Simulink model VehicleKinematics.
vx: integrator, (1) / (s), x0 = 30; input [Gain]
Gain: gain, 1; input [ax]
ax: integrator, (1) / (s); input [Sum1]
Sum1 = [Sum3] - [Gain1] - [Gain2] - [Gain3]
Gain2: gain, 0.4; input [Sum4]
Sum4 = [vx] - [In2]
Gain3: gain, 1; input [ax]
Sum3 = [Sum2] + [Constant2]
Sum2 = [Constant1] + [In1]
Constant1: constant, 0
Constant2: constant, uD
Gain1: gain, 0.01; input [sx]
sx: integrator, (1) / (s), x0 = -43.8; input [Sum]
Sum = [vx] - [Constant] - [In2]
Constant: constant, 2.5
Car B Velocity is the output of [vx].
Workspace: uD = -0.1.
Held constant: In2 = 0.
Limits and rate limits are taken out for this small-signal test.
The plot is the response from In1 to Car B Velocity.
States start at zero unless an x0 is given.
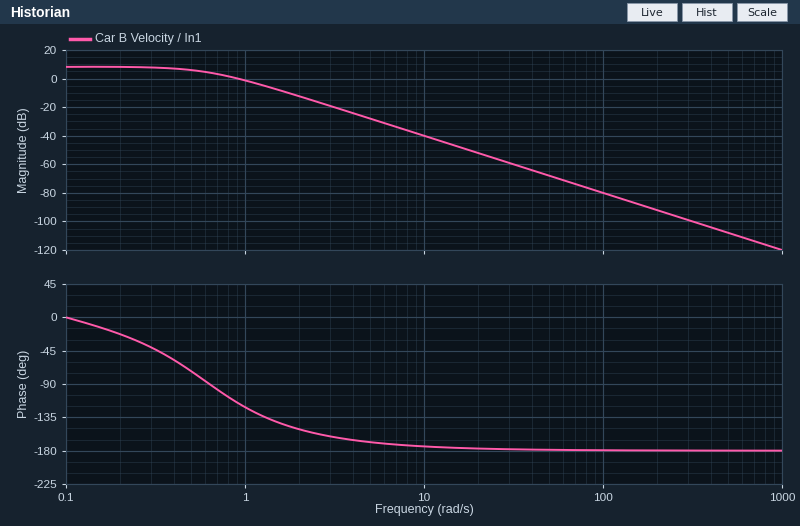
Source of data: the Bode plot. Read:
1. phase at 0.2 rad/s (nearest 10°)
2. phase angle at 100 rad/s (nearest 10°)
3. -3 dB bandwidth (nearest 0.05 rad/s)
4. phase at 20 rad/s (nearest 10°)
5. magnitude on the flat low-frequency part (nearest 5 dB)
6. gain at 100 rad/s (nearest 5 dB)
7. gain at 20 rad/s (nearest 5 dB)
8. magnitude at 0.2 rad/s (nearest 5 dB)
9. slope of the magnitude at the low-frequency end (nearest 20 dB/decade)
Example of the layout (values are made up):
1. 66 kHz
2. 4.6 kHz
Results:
1. -20°
2. -180°
3. 0.55 rad/s
4. -180°
5. 10 dB
6. -80 dB
7. -50 dB
8. 10 dB
9. 0 dB/decade
